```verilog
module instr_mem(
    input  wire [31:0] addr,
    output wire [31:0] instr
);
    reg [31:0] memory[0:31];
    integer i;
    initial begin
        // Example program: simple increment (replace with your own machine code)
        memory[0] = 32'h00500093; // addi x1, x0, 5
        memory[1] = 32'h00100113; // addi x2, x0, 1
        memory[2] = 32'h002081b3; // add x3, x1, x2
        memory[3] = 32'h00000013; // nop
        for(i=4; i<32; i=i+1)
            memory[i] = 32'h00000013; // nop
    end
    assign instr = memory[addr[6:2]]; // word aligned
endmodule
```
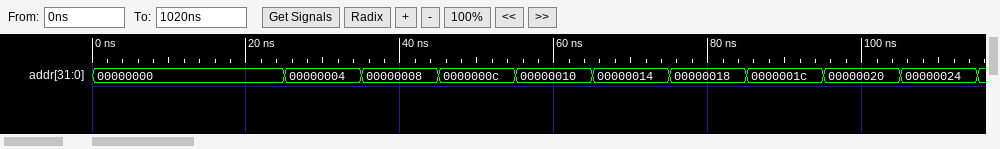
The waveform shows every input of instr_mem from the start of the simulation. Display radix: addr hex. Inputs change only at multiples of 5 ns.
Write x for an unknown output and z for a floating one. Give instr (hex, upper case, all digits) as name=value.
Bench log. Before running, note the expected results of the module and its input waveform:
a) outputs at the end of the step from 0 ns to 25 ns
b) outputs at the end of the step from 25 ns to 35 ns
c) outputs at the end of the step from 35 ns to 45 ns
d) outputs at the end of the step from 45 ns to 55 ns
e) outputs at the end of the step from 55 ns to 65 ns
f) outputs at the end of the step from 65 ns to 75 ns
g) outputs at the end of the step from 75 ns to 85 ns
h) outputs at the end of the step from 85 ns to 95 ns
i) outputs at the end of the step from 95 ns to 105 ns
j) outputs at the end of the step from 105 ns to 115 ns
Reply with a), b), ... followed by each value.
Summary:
a) instr=00500093
b) instr=00100113
c) instr=002081B3
d) instr=00000013
e) instr=00000013
f) instr=00000013
g) instr=00000013
h) instr=00000013
i) instr=00000013
j) instr=00000013
